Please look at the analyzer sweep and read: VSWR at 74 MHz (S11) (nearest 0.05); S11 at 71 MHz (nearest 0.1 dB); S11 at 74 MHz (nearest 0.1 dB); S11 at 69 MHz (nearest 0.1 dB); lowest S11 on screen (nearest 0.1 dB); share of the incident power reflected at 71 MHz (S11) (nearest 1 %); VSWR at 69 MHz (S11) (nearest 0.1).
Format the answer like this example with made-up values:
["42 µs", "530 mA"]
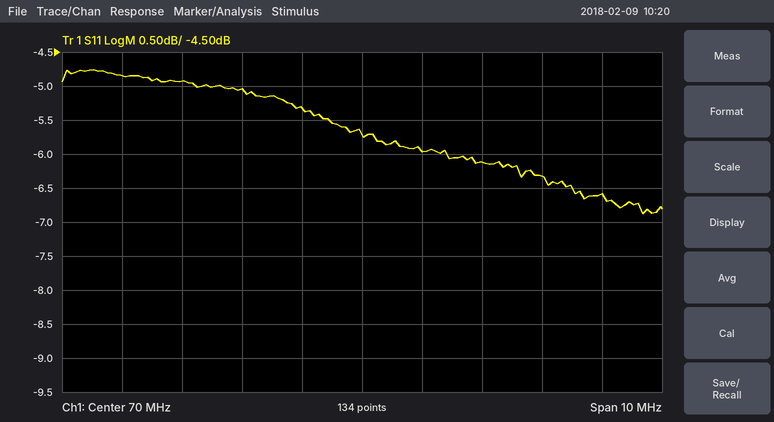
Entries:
["2.75", "-6.0 dB", "-6.6 dB", "-5.3 dB", "-6.9 dB", "25 %", "3.4"]
